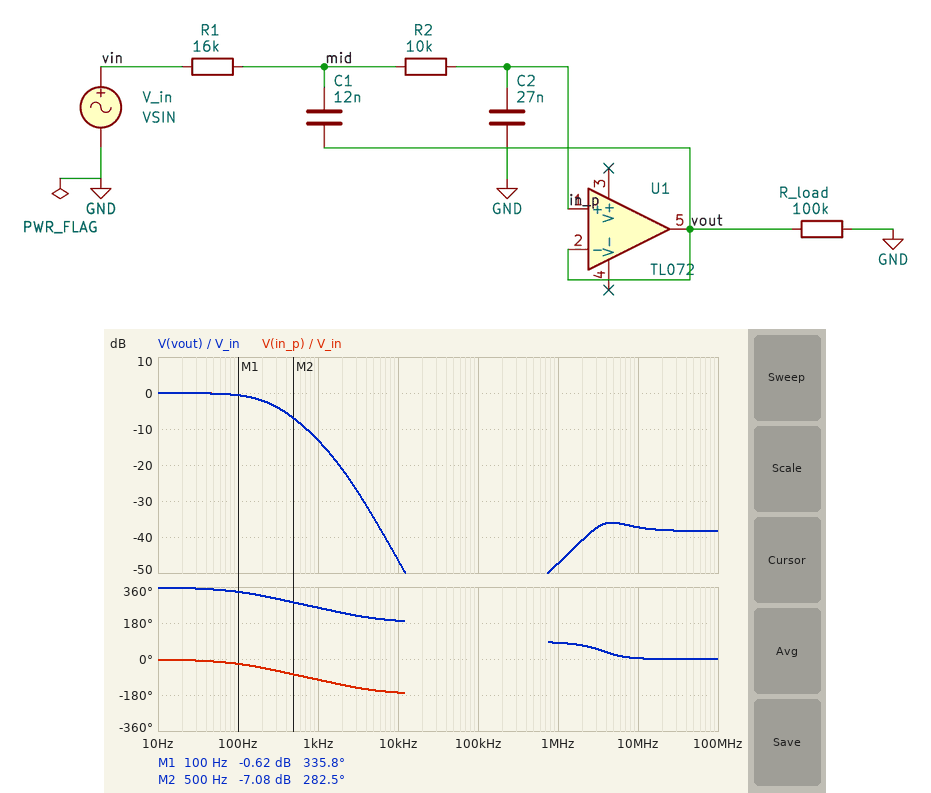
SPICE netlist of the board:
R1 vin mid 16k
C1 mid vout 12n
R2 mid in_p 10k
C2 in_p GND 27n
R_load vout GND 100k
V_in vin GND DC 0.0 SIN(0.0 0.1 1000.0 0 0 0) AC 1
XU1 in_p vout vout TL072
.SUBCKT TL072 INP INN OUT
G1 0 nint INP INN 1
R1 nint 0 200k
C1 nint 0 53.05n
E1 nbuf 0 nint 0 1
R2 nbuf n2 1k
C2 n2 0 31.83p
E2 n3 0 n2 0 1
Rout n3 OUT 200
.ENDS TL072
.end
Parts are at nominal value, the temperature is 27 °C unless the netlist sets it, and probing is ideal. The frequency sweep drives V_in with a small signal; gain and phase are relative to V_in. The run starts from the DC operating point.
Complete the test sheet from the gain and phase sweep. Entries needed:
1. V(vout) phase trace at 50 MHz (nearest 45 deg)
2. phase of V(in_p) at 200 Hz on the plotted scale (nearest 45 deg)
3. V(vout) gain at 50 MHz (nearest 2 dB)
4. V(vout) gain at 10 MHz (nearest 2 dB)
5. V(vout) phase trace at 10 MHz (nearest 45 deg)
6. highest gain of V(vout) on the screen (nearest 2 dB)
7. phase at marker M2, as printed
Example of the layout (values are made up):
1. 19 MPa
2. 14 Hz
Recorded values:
1. 0 deg
2. -45 deg
3. -38 dB
4. -38 dB
5. 0 deg
6. 0 dB
7. 282.5 deg
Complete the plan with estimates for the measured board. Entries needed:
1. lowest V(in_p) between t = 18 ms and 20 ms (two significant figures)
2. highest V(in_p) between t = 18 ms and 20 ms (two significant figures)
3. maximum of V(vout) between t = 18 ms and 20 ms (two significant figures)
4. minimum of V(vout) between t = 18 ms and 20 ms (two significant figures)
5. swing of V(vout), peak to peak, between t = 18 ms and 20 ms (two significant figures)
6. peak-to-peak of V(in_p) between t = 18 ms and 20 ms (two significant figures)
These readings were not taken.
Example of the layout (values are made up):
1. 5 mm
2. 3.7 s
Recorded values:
1. -22 mV
2. 22 mV
3. 22 mV
4. -22 mV
5. 44 mV
6. 44 mV
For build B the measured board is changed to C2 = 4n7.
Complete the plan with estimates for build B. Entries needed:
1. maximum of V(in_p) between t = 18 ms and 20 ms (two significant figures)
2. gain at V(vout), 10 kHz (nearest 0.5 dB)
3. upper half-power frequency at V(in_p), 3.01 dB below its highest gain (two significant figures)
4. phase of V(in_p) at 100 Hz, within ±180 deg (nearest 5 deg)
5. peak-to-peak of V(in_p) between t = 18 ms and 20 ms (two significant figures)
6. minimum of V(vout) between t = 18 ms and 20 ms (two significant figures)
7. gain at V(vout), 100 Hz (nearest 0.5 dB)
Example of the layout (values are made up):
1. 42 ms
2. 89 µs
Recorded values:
1. 100 mV
2. -31.0 dB
3. 1.8 kHz
4. -5 deg
5. 200 mV
6. -100 mV
7. 0 dB
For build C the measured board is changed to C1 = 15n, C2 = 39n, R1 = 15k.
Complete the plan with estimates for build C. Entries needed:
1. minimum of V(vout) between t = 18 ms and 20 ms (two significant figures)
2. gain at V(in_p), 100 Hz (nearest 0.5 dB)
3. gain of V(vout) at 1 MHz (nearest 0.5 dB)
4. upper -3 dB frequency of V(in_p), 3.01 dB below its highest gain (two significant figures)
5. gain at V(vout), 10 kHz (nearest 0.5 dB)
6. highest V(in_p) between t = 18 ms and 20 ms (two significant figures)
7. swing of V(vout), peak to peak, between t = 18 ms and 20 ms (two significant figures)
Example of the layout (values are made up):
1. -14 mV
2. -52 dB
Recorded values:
1. -15 mV
2. -1.0 dB
3. -47.0 dB
4. 180 Hz
5. -51.0 dB
6. 15 mV
7. 30 mV
